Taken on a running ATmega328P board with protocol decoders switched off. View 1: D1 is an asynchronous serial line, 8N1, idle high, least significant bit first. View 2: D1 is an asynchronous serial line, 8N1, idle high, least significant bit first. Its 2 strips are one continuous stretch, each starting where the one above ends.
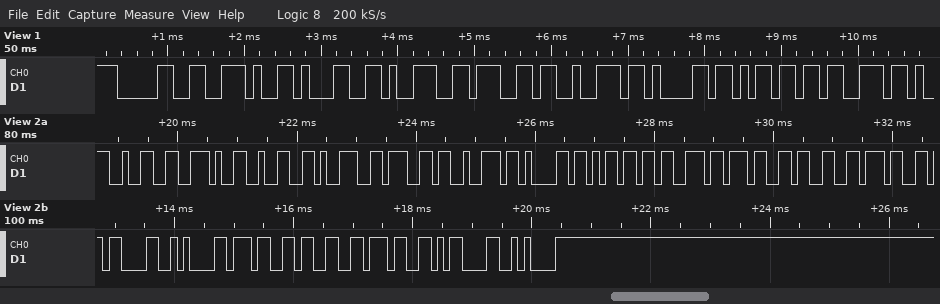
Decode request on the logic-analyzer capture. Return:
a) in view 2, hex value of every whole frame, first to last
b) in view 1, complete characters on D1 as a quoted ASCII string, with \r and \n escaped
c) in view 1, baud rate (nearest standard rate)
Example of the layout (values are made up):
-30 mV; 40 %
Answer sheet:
0x32 0x2E 0x32 0x39 0x67 0x72 0x61 0x6D 0x73 0x37 0x33 0x37 0x0D 0x0A 0x37 0x33 0x37 0x0D 0x0A; "0.19grams"; 9600 baud
